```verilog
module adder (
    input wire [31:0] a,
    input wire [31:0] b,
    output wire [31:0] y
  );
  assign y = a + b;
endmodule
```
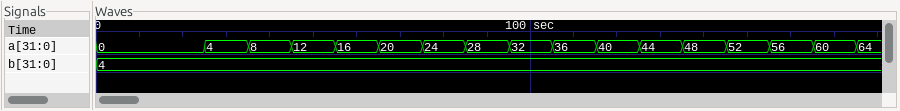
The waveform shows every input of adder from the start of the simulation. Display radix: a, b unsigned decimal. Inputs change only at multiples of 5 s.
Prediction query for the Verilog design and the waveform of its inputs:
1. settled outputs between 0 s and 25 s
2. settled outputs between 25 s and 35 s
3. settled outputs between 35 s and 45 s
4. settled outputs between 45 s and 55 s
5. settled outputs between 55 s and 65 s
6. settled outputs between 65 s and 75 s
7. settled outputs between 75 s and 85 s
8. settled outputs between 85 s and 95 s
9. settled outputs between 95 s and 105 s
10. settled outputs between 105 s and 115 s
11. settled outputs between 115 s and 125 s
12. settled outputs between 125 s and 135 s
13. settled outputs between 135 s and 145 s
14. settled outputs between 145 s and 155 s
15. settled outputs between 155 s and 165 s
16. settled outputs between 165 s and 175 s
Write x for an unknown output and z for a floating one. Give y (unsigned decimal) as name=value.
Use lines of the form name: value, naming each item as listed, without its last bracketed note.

settled outputs between 0 s and 25 s: y=4
settled outputs between 25 s and 35 s: y=8
settled outputs between 35 s and 45 s: y=12
settled outputs between 45 s and 55 s: y=16
settled outputs between 55 s and 65 s: y=20
settled outputs between 65 s and 75 s: y=24
settled outputs between 75 s and 85 s: y=28
settled outputs between 85 s and 95 s: y=32
settled outputs between 95 s and 105 s: y=36
settled outputs between 105 s and 115 s: y=40
settled outputs between 115 s and 125 s: y=44
settled outputs between 125 s and 135 s: y=48
settled outputs between 135 s and 145 s: y=52
settled outputs between 145 s and 155 s: y=56
settled outputs between 155 s and 165 s: y=60
settled outputs between 165 s and 175 s: y=64
